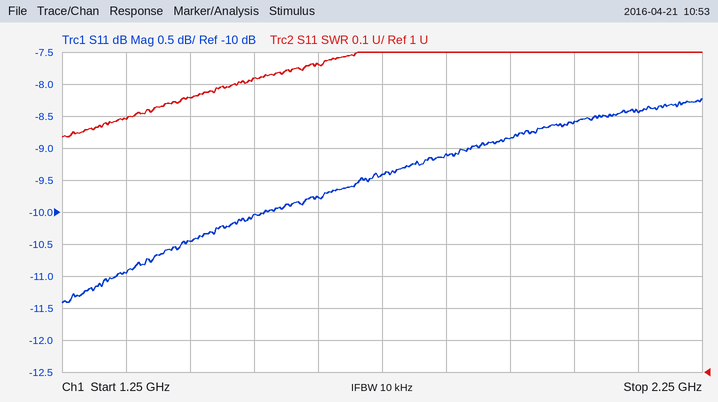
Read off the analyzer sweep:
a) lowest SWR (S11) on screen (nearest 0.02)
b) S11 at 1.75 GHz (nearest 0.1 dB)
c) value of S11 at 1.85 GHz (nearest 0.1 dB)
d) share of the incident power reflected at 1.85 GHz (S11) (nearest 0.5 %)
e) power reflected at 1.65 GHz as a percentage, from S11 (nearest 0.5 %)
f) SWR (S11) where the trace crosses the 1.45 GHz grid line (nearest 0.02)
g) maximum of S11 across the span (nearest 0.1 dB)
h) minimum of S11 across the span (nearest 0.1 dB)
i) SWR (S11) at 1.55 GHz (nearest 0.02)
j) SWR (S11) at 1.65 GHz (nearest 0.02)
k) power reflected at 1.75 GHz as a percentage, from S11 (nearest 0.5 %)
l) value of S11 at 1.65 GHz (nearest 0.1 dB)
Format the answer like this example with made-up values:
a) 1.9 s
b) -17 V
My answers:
a) 1.74
b) -9.4 dB
c) -9.1 dB
d) 12.5 %
e) 10.5 %
f) 1.86
g) -8.2 dB
h) -11.4 dB
i) 1.92
j) 1.96
k) 11.5 %
l) -9.8 dB
